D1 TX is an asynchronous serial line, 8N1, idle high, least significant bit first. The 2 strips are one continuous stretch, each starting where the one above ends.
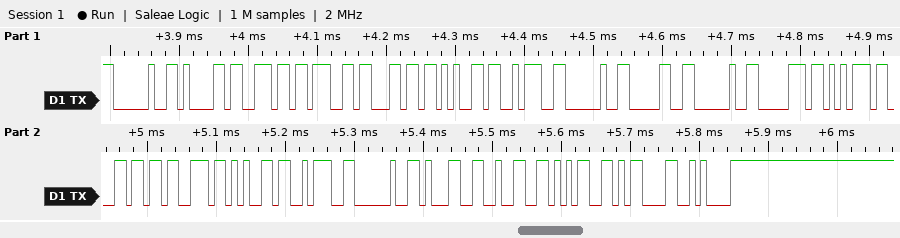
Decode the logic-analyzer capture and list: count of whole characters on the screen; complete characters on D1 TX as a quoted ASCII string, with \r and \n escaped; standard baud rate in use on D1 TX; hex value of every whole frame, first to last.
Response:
22
" angle: 0 pulse: 125\r\n"
115200 baud
20 61 6E 67 6C 65 3A 20 30 20 70 75 6C 73 65 3A 20 31 32 35 0D 0A
